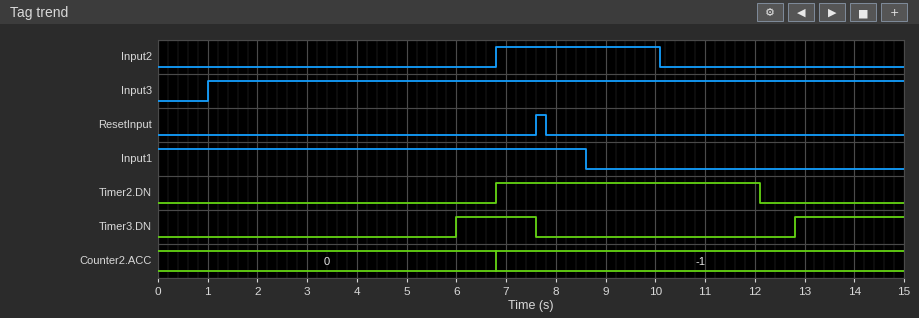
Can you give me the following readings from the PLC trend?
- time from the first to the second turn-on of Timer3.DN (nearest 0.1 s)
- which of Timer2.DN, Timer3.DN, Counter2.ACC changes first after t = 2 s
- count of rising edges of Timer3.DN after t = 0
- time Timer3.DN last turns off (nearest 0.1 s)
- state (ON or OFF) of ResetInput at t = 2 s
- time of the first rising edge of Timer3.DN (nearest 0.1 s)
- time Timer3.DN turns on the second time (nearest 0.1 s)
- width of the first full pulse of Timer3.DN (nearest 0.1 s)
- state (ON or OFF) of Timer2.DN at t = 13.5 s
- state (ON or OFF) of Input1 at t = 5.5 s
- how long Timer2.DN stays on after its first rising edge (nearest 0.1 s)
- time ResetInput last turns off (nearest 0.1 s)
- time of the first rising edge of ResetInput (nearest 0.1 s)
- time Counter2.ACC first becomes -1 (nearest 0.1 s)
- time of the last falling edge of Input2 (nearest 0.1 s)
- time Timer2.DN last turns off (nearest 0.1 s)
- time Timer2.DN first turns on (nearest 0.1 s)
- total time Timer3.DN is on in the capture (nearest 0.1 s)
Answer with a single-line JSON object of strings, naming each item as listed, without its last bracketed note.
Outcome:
{"time from the first to the second turn-on of Timer3.DN": "6.8 s", "which of Timer2.DN, Timer3.DN, Counter2.ACC changes first after t = 2 s": "Timer3.DN", "count of rising edges of Timer3.DN after t = 0": "2", "time Timer3.DN last turns off": "7.6 s", "state (ON or OFF) of ResetInput at t = 2 s": "OFF", "time of the first rising edge of Timer3.DN": "6.0 s", "time Timer3.DN turns on the second time": "12.8 s", "width of the first full pulse of Timer3.DN": "1.6 s", "state (ON or OFF) of Timer2.DN at t = 13.5 s": "OFF", "state (ON or OFF) of Input1 at t = 5.5 s": "ON", "how long Timer2.DN stays on after its first rising edge": "5.3 s", "time ResetInput last turns off": "7.8 s", "time of the first rising edge of ResetInput": "7.6 s", "time Counter2.ACC first becomes -1": "6.8 s", "time of the last falling edge of Input2": "10.1 s", "time Timer2.DN last turns off": "12.1 s", "time Timer2.DN first turns on": "6.8 s", "total time Timer3.DN is on in the capture": "3.8 s"}
